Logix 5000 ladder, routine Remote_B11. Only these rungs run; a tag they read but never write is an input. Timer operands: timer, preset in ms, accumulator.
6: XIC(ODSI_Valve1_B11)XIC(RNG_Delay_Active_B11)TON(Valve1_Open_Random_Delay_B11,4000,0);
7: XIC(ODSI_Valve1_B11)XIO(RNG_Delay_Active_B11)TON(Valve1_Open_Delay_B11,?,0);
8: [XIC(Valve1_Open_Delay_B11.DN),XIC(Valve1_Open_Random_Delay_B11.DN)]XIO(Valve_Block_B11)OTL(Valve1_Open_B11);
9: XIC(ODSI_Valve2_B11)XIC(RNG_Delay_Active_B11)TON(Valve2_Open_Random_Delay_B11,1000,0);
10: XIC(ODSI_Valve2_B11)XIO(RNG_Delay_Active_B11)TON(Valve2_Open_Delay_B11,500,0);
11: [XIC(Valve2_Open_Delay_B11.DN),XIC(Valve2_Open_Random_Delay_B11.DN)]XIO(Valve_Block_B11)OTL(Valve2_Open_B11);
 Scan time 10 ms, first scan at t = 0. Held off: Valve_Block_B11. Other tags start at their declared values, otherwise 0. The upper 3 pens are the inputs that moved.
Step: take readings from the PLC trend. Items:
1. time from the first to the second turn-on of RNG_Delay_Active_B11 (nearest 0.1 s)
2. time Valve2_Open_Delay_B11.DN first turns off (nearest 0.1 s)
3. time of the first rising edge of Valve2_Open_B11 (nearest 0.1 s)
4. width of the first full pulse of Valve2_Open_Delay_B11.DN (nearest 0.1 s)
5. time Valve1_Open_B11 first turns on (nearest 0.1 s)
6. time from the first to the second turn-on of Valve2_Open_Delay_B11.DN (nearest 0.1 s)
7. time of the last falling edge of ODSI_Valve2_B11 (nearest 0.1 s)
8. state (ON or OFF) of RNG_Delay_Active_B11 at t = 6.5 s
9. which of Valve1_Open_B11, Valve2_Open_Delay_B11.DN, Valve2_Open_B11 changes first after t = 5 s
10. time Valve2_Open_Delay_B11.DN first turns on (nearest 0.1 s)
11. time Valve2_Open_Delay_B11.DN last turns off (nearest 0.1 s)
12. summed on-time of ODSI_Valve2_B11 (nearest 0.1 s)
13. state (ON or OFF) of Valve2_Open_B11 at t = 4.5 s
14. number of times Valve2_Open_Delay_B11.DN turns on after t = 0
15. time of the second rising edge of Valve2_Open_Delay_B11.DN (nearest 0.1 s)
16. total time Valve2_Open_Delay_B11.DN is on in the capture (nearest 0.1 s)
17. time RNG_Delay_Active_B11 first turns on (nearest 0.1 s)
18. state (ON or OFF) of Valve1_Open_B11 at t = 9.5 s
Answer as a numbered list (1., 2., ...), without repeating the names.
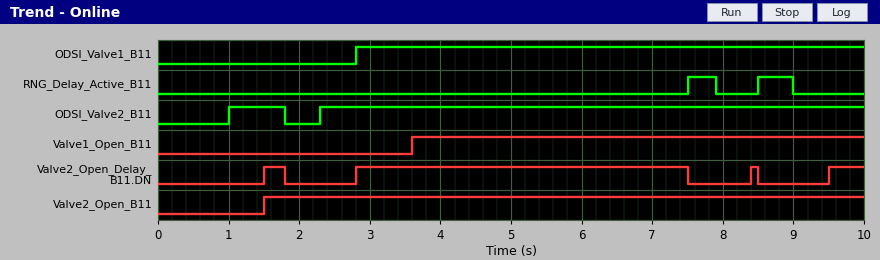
1. 1.0 s
2. 1.8 s
3. 1.5 s
4. 0.3 s
5. 3.6 s
6. 1.3 s
7. 1.8 s
8. OFF
9. Valve2_Open_Delay_B11.DN
10. 1.5 s
11. 8.5 s
12. 8.5 s
13. ON
14. 4
15. 2.8 s
16. 5.6 s
17. 7.5 s
18. ON
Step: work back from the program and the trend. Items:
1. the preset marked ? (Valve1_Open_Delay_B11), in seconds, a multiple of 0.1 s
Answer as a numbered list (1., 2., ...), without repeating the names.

1. 0.8 s
